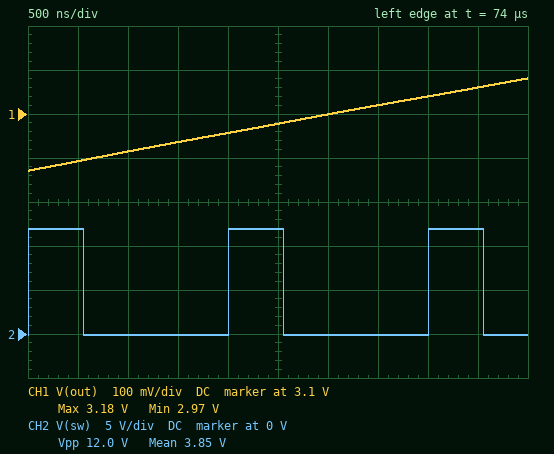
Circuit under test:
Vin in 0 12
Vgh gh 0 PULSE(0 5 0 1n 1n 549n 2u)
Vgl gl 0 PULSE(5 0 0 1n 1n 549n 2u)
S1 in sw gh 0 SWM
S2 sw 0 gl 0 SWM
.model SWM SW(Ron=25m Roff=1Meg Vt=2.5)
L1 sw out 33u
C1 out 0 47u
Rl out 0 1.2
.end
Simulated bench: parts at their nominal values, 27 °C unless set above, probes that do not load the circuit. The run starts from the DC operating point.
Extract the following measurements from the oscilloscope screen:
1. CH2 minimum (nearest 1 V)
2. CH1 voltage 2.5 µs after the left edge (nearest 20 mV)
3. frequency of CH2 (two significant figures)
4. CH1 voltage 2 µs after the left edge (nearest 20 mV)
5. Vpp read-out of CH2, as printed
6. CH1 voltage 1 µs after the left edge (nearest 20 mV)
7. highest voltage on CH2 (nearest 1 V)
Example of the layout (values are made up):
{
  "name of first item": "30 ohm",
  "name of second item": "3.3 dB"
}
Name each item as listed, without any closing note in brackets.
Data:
{
  "CH2 minimum": "0 V",
  "CH1 voltage 2.5 µs after the left edge": "3.08 V",
  "frequency of CH2": "500 kHz",
  "CH1 voltage 2 µs after the left edge": "3.06 V",
  "Vpp read-out of CH2, as printed": "12.0 V",
  "CH1 voltage 1 µs after the left edge": "3.02 V",
  "highest voltage on CH2": "12 V"
}
